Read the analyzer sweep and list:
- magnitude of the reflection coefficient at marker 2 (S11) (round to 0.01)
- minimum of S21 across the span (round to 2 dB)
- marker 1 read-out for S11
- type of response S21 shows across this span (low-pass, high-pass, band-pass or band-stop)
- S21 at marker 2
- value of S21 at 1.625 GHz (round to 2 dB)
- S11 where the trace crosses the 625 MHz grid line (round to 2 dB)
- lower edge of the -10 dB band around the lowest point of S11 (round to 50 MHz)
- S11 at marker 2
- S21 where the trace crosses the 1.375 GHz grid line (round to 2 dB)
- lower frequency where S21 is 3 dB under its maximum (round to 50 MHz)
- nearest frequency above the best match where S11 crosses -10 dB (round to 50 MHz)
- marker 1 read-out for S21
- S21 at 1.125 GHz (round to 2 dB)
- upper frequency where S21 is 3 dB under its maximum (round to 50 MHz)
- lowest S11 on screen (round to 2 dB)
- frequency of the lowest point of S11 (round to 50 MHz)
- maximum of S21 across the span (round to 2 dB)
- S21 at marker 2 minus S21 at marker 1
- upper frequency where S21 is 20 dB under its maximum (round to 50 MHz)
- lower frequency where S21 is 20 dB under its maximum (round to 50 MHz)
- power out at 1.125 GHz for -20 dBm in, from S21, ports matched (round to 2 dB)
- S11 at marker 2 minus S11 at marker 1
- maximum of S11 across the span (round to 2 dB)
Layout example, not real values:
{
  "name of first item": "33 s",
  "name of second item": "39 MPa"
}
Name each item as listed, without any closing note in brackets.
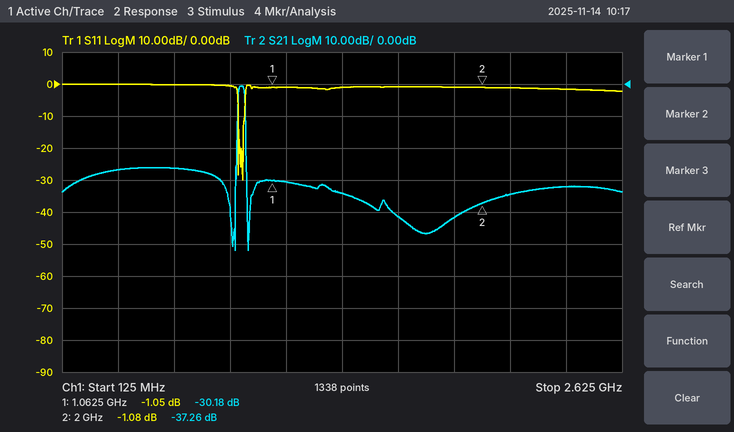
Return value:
{
  "magnitude of the reflection coefficient at marker 2 (S11)": "0.88",
  "minimum of S21 across the span": "-52 dB",
  "marker 1 read-out for S11": "-1.05 dB",
  "type of response S21 shows across this span": "band-pass",
  "S21 at marker 2": "-37.26 dB",
  "value of S21 at 1.625 GHz": "-42 dB",
  "S11 where the trace crosses the 625 MHz grid line": "0 dB",
  "lower edge of the -10 dB band around the lowest point of S11": "900 MHz",
  "S11 at marker 2": "-1.08 dB",
  "S21 where the trace crosses the 1.375 GHz grid line": "-34 dB",
  "lower frequency where S21 is 3 dB under its maximum": "900 MHz",
  "nearest frequency above the best match where S11 crosses -10 dB": "950 MHz",
  "marker 1 read-out for S21": "-30.18 dB",
  "S21 at 1.125 GHz": "-30 dB",
  "upper frequency where S21 is 3 dB under its maximum": "950 MHz",
  "lowest S11 on screen": "-30 dB",
  "frequency of the lowest point of S11": "950 MHz",
  "maximum of S21 across the span": "0 dB",
  "S21 at marker 2 minus S21 at marker 1": "-7.08 dB",
  "upper frequency where S21 is 20 dB under its maximum": "950 MHz",
  "lower frequency where S21 is 20 dB under its maximum": "900 MHz",
  "power out at 1.125 GHz for -20 dBm in, from S21, ports matched": "-50 dBm",
  "S11 at marker 2 minus S11 at marker 1": "-0.03 dB",
  "maximum of S11 across the span": "0 dB"
}
